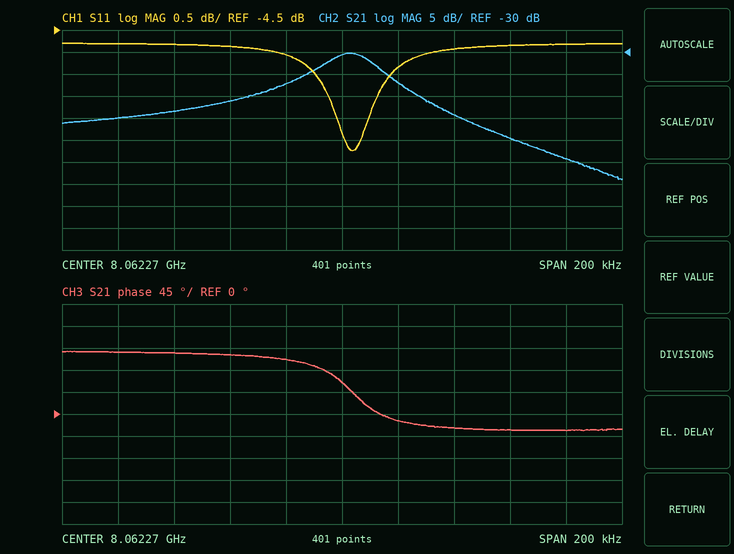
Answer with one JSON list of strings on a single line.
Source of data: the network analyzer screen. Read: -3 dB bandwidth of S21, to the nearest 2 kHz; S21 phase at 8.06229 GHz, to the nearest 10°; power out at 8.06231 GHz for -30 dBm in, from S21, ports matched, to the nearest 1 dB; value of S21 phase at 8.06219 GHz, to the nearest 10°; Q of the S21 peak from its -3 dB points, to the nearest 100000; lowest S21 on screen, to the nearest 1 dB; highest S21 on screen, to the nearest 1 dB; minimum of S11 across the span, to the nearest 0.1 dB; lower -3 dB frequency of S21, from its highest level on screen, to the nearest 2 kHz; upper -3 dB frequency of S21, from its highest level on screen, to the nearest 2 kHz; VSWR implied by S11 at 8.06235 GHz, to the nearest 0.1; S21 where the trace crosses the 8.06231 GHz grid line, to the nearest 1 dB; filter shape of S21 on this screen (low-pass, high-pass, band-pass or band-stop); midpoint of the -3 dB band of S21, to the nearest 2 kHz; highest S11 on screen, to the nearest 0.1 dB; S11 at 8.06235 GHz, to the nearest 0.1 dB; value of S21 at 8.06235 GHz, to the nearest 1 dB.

["20 kHz", "-10°", "-74 dBm", "130°", "400000", "-59 dB", "-30 dB", "-7.2 dB", "8.062262 GHz", "8.062282 GHz", "3.7", "-44 dB", "band-pass", "8.062272 GHz", "-4.8 dB", "-4.8 dB", "-54 dB"]
